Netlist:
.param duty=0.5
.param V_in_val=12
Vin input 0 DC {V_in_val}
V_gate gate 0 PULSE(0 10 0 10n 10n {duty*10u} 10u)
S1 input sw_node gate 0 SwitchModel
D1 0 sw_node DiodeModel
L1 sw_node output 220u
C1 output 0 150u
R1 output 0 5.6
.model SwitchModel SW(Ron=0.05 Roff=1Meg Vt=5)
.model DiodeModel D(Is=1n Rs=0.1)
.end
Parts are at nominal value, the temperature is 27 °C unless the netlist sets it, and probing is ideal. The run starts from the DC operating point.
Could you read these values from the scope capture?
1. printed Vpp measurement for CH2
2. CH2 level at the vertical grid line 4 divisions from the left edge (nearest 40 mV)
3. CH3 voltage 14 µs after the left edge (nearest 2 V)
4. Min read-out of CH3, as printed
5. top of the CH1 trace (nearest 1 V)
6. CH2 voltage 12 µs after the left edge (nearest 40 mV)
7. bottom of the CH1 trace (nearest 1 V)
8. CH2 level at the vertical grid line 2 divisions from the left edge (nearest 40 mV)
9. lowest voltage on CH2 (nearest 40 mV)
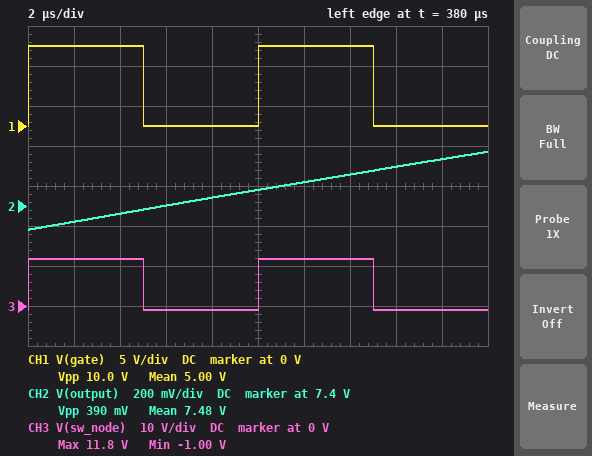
390 mV
7.44 V
12 V
-1.00 V
10 V
7.52 V
0 V
7.36 V
7.28 V
